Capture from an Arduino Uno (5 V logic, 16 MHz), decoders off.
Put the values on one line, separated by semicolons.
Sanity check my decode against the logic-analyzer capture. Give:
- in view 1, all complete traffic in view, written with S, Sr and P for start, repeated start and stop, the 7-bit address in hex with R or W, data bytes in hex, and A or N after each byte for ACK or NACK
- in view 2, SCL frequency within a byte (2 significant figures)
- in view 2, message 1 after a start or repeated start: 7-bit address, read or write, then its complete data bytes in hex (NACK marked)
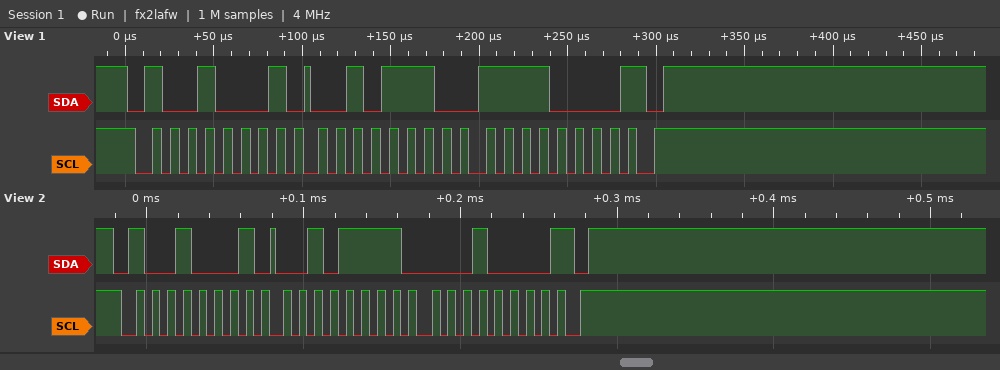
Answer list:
S 48R A 2E A F0 N P; 100 kHz; 0x48 read: 2F 10 NACK
